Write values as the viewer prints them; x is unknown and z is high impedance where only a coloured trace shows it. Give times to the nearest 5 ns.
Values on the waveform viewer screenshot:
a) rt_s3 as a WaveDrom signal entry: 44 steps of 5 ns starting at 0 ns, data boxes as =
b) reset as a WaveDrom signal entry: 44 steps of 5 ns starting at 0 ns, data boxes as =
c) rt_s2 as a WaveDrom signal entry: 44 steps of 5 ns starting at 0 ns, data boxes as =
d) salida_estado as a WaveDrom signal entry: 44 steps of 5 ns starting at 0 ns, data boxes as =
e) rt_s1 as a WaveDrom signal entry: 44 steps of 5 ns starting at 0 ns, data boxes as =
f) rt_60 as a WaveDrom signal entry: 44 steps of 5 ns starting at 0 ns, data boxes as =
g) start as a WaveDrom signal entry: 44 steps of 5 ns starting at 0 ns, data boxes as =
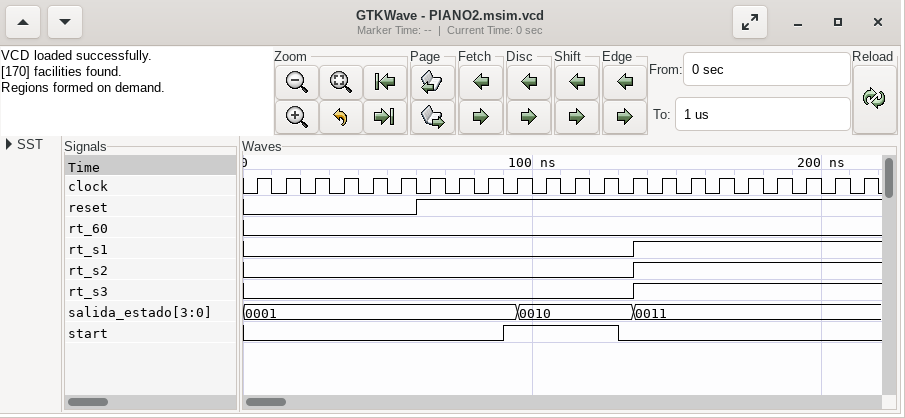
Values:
{name: 'rt_s3', wave: '0..........................1................'}
{name: 'reset', wave: '0...........1...............................'}
{name: 'rt_s2', wave: '0..........................1................'}
{name: 'salida_estado', wave: '=..................=.......=................', data: '0001 0010 0011'}
{name: 'rt_s1', wave: '0..........................1................'}
{name: 'rt_60', wave: '0...........................................'}
{name: 'start', wave: '0.................1.......0.................'}
